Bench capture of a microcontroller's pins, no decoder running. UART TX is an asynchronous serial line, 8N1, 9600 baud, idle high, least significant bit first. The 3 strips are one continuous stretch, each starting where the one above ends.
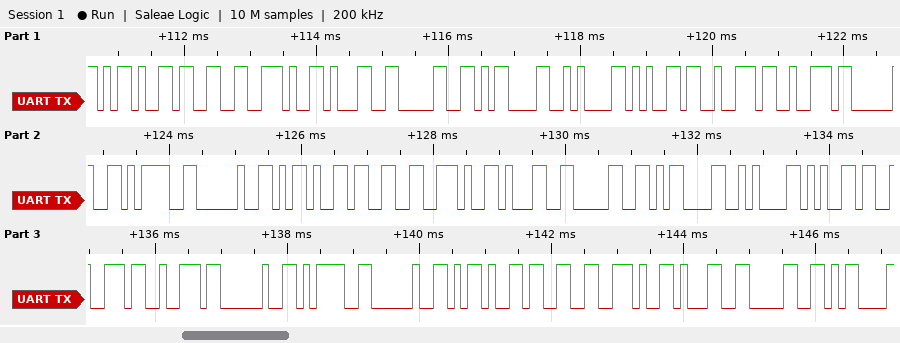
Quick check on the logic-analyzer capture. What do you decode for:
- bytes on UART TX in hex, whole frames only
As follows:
2D 33 2E 31 30 0D 0A 65 72 72 20 3D 20 2D 33 2E 31 30 0D 0A 65 72 72 20 3D 20 2D 33 2E 31 30 0D
